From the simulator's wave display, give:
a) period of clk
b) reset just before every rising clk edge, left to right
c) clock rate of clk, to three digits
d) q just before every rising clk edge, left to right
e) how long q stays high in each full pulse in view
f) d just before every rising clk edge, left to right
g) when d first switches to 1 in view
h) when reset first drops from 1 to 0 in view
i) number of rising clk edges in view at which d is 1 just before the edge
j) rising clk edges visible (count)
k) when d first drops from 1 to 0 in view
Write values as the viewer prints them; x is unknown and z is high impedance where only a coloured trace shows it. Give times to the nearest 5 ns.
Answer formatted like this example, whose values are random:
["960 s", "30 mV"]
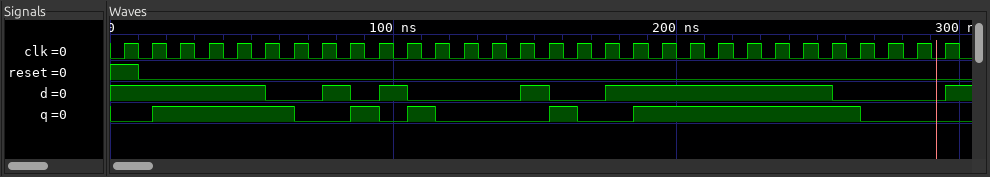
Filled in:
["10 ns", "1 0 0 0 0 0 0 0 0 0 0 0 0 0 0 0 0 0 0 0 0 0 0 0 0 0 0 0 0 0", "100 MHz", "0 0 1 1 1 1 1 0 0 1 0 1 0 0 0 0 1 0 0 1 1 1 1 1 1 1 1 0 0 0", "50 ns, 10 ns, 10 ns, 10 ns, 80 ns", "1 1 1 1 1 1 0 0 1 0 1 0 0 0 0 1 0 0 1 1 1 1 1 1 1 1 0 0 0 0", "75 ns", "10 ns", "17", "30", "55 ns"]
